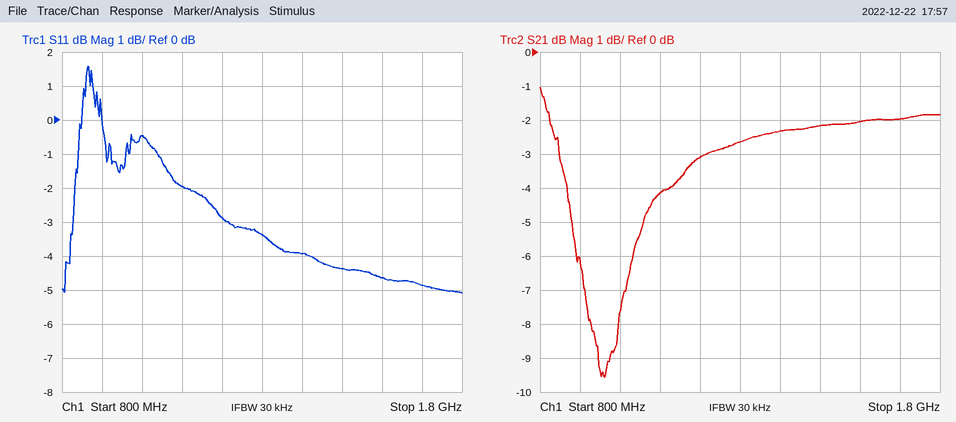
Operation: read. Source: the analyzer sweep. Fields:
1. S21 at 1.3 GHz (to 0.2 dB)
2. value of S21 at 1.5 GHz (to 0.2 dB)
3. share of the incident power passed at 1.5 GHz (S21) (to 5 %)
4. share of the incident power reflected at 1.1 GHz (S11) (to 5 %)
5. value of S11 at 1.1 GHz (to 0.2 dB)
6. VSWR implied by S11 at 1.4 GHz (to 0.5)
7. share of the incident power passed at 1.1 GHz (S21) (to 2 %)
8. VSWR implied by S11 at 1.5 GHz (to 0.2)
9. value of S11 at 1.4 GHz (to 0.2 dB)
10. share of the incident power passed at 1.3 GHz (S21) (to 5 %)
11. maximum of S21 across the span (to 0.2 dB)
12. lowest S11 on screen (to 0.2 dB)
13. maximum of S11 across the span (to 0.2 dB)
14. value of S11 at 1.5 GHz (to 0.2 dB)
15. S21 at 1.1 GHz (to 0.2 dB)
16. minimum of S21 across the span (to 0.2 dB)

-2.6 dB
-2.2 dB
60 %
65 %
-2.0 dB
4.5
38 %
4.0
-4.0 dB
55 %
-1.0 dB
-5.0 dB
1.6 dB
-4.4 dB
-4.2 dB
-9.6 dB
